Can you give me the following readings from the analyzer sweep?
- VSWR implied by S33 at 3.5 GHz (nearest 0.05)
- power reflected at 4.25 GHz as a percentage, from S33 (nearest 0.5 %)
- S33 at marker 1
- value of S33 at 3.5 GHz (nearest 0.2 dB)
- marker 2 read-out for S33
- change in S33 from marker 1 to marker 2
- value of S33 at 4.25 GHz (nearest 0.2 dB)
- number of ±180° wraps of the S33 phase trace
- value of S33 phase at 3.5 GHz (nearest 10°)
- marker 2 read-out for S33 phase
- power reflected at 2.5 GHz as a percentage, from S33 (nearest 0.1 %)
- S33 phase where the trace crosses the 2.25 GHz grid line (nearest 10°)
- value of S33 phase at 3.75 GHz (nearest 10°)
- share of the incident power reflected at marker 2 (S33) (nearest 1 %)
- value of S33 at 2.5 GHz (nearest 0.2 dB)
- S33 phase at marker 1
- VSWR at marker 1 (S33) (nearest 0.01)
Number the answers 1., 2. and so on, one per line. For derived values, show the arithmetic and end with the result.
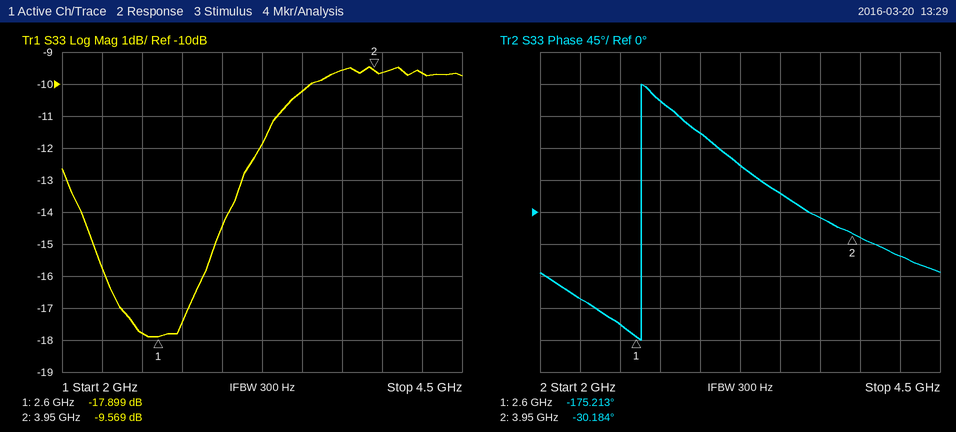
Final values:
1. |Γ| = 10^(-10.2/20) = 0.3090; VSWR = (1 + 0.3090)/(1 − 0.3090) ≈ 1.89, so 1.90 to the nearest 0.05
2. 10^(-9.6/10) ≈ 11.0 %
3. -17.899 dB
4. -10.2 dB
5. -9.569 dB
6. -9.569 − (-17.899) = 8.330 dB
7. -9.6 dB
8. 1
9. 30°
10. -30.184°
11. 10^(-17.8/10) ≈ 1.7 %
12. -120°
13. -10°
14. 10^(-9.569/10) ≈ 11 %
15. -17.8 dB
16. -175.213°
17. (1 + 0.1274)/(1 − 0.1274) ≈ 1.29
